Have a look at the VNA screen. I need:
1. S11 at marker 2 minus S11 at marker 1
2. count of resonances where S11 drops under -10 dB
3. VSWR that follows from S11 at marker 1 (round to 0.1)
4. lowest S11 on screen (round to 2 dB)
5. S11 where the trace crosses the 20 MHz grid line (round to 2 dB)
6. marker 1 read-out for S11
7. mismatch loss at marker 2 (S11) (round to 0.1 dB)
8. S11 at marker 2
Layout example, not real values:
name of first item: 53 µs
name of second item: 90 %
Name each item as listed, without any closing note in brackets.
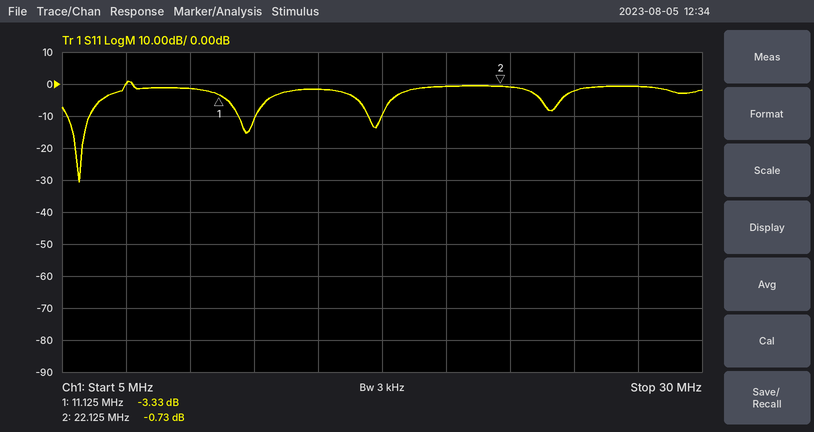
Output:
S11 at marker 2 minus S11 at marker 1: 2.60 dB
count of resonances where S11 drops under -10 dB: 3
VSWR that follows from S11 at marker 1: 5.3
lowest S11 on screen: -30 dB
S11 where the trace crosses the 20 MHz grid line: 0 dB
marker 1 read-out for S11: -3.33 dB
mismatch loss at marker 2 (S11): 8.1 dB
S11 at marker 2: -0.73 dB
